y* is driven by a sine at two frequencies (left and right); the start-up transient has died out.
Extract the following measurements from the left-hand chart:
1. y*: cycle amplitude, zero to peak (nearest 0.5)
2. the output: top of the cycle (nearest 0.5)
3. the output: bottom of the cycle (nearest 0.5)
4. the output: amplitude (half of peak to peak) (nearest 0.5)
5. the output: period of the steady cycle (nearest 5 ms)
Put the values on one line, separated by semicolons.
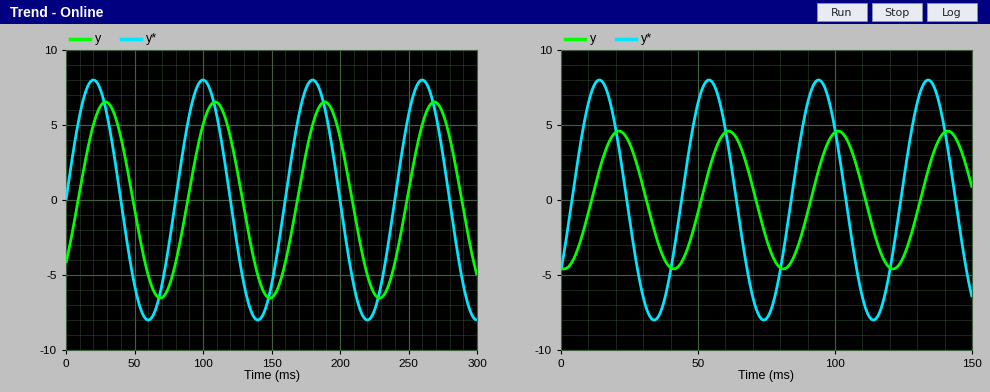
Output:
8.0; 6.5; -6.5; 6.5; 80 ms
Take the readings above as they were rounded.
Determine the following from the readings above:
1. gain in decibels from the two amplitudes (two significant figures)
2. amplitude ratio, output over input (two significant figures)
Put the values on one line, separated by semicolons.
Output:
-1.8 dB; 0.81
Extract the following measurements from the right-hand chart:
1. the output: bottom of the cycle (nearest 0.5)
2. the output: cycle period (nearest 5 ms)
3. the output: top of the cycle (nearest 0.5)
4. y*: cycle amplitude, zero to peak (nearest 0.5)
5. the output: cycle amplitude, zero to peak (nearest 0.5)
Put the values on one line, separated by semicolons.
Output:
-4.5; 40 ms; 4.5; 8.0; 4.5
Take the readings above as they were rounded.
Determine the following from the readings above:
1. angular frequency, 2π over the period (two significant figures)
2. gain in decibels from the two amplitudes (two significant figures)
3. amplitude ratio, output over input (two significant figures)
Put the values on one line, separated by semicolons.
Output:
0.16 rad/ms; -5.0 dB; 0.56
